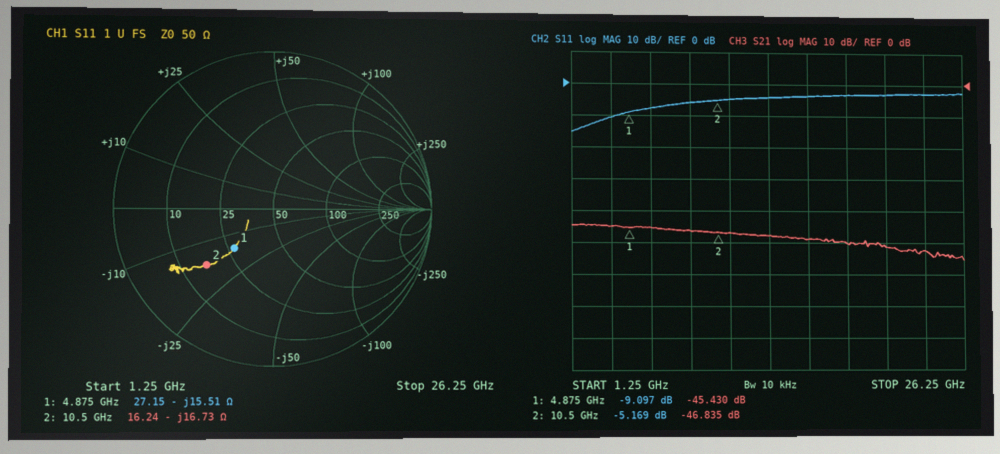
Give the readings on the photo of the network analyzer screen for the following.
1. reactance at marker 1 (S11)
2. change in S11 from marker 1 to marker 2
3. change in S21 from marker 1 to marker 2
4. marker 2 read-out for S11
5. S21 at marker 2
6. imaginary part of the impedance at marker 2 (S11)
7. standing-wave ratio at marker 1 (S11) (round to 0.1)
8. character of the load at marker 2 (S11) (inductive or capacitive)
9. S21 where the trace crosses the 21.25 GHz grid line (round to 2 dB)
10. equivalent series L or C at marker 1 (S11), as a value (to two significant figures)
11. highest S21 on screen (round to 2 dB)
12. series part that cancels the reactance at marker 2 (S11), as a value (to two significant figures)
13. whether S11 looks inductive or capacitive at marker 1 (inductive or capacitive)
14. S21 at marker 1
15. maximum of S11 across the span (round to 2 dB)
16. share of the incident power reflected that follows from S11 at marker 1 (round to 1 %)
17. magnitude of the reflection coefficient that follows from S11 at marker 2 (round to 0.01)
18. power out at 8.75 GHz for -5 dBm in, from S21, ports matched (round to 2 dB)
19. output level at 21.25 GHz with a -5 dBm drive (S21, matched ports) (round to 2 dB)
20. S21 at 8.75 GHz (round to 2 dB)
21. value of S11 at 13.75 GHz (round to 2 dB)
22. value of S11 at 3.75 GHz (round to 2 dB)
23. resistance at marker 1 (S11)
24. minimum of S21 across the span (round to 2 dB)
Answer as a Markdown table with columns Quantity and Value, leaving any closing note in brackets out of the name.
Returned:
| Quantity | Value |
|---|---|
| reactance at marker 1 | -15.51 Ω |
| change in S11 from marker 1 to marker 2 | 3.928 dB |
| change in S21 from marker 1 to marker 2 | -1.405 dB |
| marker 2 read-out for S11 | -5.169 dB |
| S21 at marker 2 | -46.835 dB |
| imaginary part of the impedance at marker 2 | -16.73 Ω |
| standing-wave ratio at marker 1 (S11) | 2.1 |
| character of the load at marker 2 (S11) | capacitive |
| S21 where the trace crosses the 21.25 GHz grid line | -52 dB |
| equivalent series L or C at marker 1 (S11), as a value | 2.1 pF |
| highest S21 on screen | -44 dB |
| series part that cancels the reactance at marker 2 (S11), as a value | 250 pH |
| whether S11 looks inductive or capacitive at marker 1 | capacitive |
| S21 at marker 1 | -45.430 dB |
| maximum of S11 across the span | -2 dB |
| share of the incident power reflected that follows from S11 at marker 1 | 12 % |
| magnitude of the reflection coefficient that follows from S11 at marker 2 | 0.55 |
| power out at 8.75 GHz for -5 dBm in, from S21, ports matched | -52 dBm |
| output level at 21.25 GHz with a -5 dBm drive (S21, matched ports) | -56 dBm |
| S21 at 8.75 GHz | -46 dB |
| value of S11 at 13.75 GHz | -4 dB |
| value of S11 at 3.75 GHz | -10 dB |
| resistance at marker 1 | 27.15 Ω |
| minimum of S21 across the span | -56 dB |
